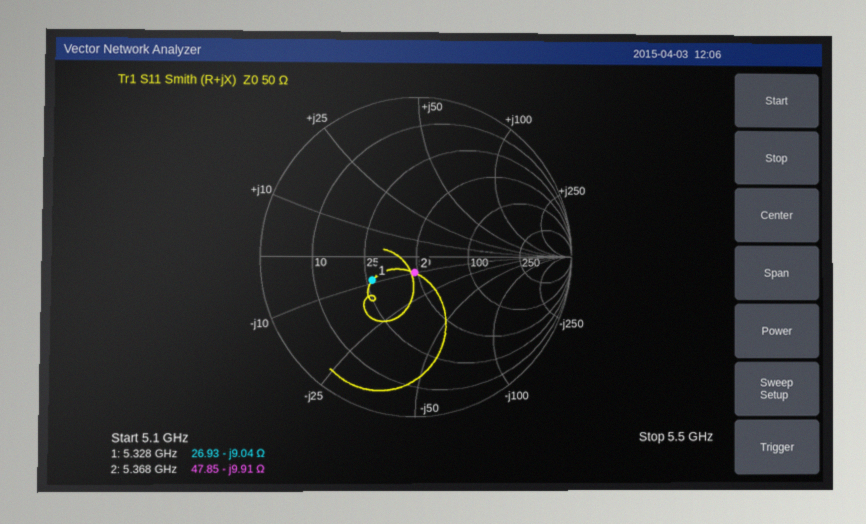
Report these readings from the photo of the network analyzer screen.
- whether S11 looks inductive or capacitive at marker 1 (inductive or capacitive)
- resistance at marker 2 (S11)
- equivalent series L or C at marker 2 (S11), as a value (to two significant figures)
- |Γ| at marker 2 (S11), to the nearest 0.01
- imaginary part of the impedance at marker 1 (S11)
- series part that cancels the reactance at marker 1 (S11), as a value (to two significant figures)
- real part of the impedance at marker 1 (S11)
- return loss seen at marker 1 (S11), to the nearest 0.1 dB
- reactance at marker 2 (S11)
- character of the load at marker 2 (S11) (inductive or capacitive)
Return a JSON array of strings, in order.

["capacitive", "47.85 Ω", "3.0 pF", "0.10", "-9.04 Ω", "270 pH", "26.93 Ω", "9.9 dB", "-9.91 Ω", "capacitive"]
